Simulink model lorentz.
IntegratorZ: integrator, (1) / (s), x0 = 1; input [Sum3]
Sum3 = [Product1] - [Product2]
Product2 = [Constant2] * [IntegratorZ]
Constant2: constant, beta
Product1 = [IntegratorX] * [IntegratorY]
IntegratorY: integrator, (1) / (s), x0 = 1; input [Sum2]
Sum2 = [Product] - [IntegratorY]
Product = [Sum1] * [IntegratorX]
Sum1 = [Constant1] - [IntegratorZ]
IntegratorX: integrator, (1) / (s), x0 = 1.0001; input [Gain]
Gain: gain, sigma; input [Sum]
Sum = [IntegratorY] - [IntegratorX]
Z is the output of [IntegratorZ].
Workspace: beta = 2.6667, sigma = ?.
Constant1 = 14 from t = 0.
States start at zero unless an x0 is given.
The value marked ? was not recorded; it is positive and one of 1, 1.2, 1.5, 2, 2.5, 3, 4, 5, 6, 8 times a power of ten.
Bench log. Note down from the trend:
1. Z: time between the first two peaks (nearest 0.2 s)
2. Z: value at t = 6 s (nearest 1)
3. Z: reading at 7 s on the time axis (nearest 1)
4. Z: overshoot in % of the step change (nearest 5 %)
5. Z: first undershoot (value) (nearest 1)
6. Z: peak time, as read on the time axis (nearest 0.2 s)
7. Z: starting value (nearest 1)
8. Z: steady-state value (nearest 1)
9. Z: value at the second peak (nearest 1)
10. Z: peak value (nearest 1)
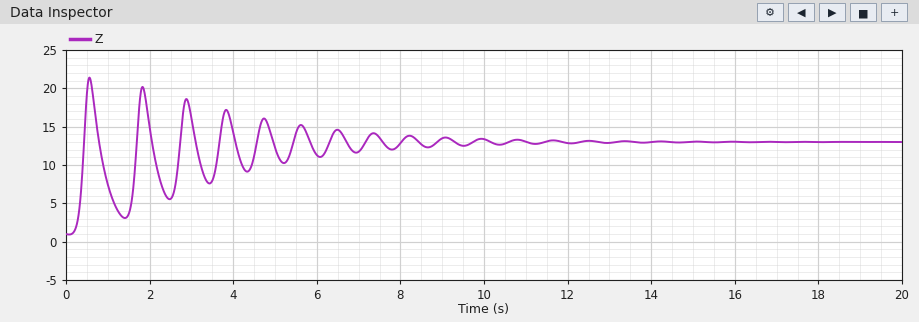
1.2 s
11
12
70 %
3
0.6 s
1
13
20
21
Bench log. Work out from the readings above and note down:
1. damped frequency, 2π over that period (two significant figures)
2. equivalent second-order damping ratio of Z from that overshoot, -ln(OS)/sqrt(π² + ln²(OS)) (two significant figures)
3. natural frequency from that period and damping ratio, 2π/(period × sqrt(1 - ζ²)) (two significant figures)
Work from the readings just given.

5.2 rad/s
0.11
5.3 rad/s
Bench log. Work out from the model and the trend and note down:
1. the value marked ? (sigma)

10
